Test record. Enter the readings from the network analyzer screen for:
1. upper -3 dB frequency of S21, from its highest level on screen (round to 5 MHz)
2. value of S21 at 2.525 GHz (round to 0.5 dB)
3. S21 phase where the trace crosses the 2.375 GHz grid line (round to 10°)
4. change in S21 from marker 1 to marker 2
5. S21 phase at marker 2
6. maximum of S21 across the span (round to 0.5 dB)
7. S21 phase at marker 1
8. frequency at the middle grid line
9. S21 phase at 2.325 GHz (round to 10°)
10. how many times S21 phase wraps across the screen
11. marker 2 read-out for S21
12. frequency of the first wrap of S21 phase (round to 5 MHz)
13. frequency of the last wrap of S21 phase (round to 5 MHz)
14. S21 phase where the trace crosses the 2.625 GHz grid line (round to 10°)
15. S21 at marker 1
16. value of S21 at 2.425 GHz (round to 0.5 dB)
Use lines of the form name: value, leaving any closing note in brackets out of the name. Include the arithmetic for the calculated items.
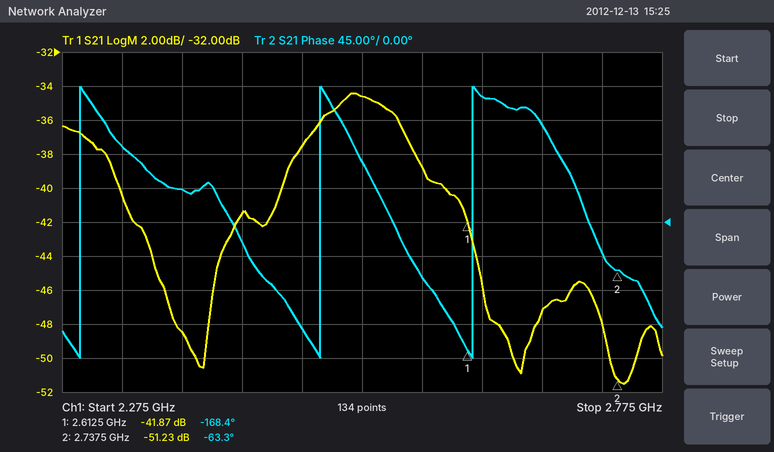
upper -3 dB frequency of S21, from its highest level on screen: 2.565 GHz
value of S21 at 2.525 GHz: -34.5 dB
S21 phase where the trace crosses the 2.375 GHz grid line: 40°
change in S21 from marker 1 to marker 2: -51.23 − (-41.87) = -9.36 dB
S21 phase at marker 2: -63.3°
maximum of S21 across the span: -34.5 dB
S21 phase at marker 1: -168.4°
frequency at the middle grid line: 2.525 GHz
S21 phase at 2.325 GHz: 100°
how many times S21 phase wraps across the screen: 3
marker 2 read-out for S21: -51.23 dB
frequency of the first wrap of S21 phase: 2.290 GHz
frequency of the last wrap of S21 phase: 2.620 GHz
S21 phase where the trace crosses the 2.625 GHz grid line: 170°
S21 at marker 1: -41.87 dB
value of S21 at 2.425 GHz: -41.5 dB
